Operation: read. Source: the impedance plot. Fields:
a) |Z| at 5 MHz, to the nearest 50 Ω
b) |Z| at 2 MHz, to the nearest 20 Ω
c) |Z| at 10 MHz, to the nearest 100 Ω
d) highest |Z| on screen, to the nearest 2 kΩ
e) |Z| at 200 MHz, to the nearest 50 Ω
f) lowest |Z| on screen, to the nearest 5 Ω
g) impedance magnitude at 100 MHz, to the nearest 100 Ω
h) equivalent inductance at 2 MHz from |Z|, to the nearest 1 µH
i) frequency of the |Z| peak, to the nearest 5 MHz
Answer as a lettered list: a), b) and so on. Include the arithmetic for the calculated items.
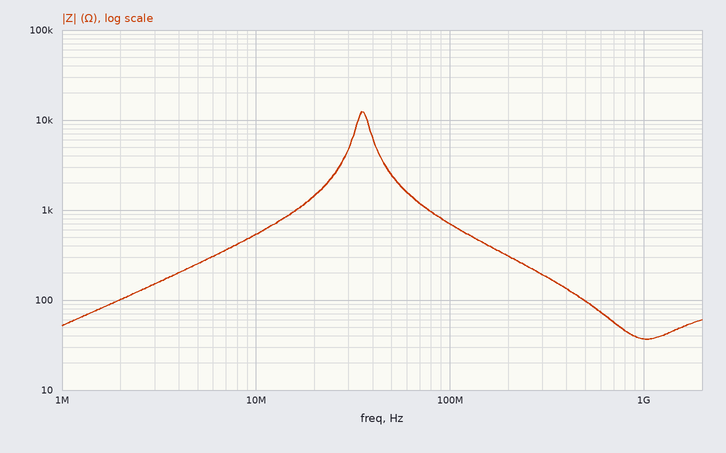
a) 250 Ω
b) 100 Ω
c) 500 Ω
d) 12 kΩ
e) 300 Ω
f) 35 Ω
g) 700 Ω
h) L = 100 Ω/(2π × 2 MHz) ≈ 8 µH
i) 35 MHz
